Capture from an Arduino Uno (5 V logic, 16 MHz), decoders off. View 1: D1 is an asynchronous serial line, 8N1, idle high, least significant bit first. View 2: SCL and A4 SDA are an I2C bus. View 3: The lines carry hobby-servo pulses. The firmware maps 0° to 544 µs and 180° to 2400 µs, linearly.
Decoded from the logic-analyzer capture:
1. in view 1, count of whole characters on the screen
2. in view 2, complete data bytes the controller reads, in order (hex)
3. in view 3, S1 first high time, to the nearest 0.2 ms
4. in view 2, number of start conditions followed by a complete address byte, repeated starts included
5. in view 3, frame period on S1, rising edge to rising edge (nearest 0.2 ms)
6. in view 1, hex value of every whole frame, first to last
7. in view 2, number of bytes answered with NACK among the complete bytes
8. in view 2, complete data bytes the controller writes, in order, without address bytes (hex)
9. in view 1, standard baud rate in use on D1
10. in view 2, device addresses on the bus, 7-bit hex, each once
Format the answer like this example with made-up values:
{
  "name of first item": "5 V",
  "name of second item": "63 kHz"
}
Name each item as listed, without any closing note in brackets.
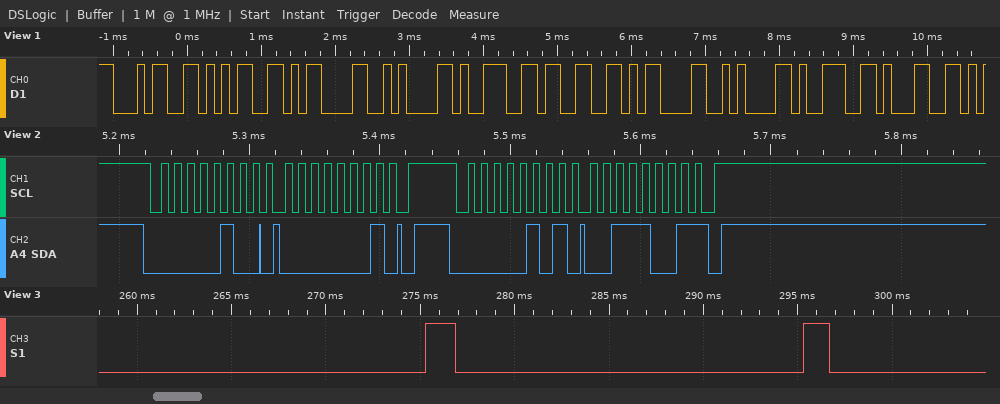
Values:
{
  "in view 1, count of whole characters on the screen": "10",
  "in view 2, complete data bytes the controller reads, in order": "39",
  "in view 3, S1 first high time, to the nearest 0.2 ms": "1.6 ms",
  "in view 2, number of start conditions followed by a complete address byte, repeated starts included": "2",
  "in view 3, frame period on S1, rising edge to rising edge": "20.0 ms",
  "in view 1, hex value of every whole frame, first to last": "34 35 0D 0A 39 33 0D 0A 39 31",
  "in view 2, number of bytes answered with NACK among the complete bytes": "1",
  "in view 2, complete data bytes the controller writes, in order, without address bytes": "01",
  "in view 1, standard baud rate in use on D1": "9600 baud",
  "in view 2, device addresses on the bus, 7-bit hex, each once": "0x02"
}
